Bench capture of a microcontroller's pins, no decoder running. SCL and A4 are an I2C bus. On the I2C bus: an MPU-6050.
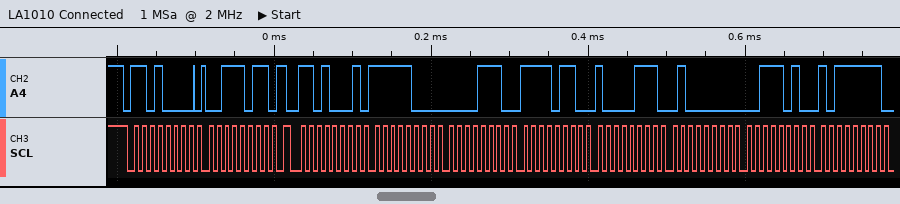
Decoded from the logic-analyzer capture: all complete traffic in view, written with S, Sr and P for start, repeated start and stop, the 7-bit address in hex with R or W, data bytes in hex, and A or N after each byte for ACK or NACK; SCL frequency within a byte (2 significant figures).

S 68W A 3B A Sr 68R A F8 A 0E A F6 A 87 A 40 A 3A A BF A
100 kHz
